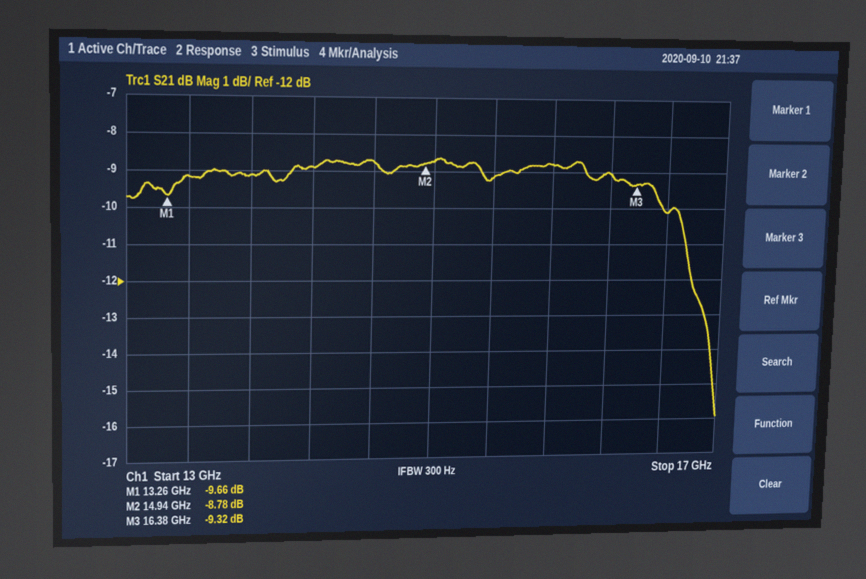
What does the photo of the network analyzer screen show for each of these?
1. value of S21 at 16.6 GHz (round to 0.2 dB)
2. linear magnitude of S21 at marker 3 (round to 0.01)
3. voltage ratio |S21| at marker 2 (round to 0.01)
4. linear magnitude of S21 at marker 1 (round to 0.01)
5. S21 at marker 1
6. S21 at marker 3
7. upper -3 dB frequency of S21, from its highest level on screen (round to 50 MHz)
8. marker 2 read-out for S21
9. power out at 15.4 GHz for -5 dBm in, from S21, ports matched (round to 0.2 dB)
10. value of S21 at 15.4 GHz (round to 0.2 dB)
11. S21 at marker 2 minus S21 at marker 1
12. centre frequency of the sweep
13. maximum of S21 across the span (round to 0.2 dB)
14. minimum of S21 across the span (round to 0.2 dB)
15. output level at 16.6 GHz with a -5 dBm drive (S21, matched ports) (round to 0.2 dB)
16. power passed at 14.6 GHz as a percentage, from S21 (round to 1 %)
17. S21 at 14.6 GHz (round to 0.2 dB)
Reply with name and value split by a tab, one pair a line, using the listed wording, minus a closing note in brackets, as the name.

value of S21 at 16.6 GHz	-10.2 dB
linear magnitude of S21 at marker 3	0.34
voltage ratio |S21| at marker 2	0.36
linear magnitude of S21 at marker 1	0.33
S21 at marker 1	-9.66 dB
S21 at marker 3	-9.32 dB
upper -3 dB frequency of S21, from its highest level on screen	16.75 GHz
marker 2 read-out for S21	-8.78 dB
power out at 15.4 GHz for -5 dBm in, from S21, ports matched	-14.2 dBm
value of S21 at 15.4 GHz	-9.2 dB
S21 at marker 2 minus S21 at marker 1	0.88 dB
centre frequency of the sweep	15 GHz
maximum of S21 across the span	-8.6 dB
minimum of S21 across the span	-16.0 dB
output level at 16.6 GHz with a -5 dBm drive (S21, matched ports)	-15.2 dBm
power passed at 14.6 GHz as a percentage, from S21	13 %
S21 at 14.6 GHz	-8.8 dB
